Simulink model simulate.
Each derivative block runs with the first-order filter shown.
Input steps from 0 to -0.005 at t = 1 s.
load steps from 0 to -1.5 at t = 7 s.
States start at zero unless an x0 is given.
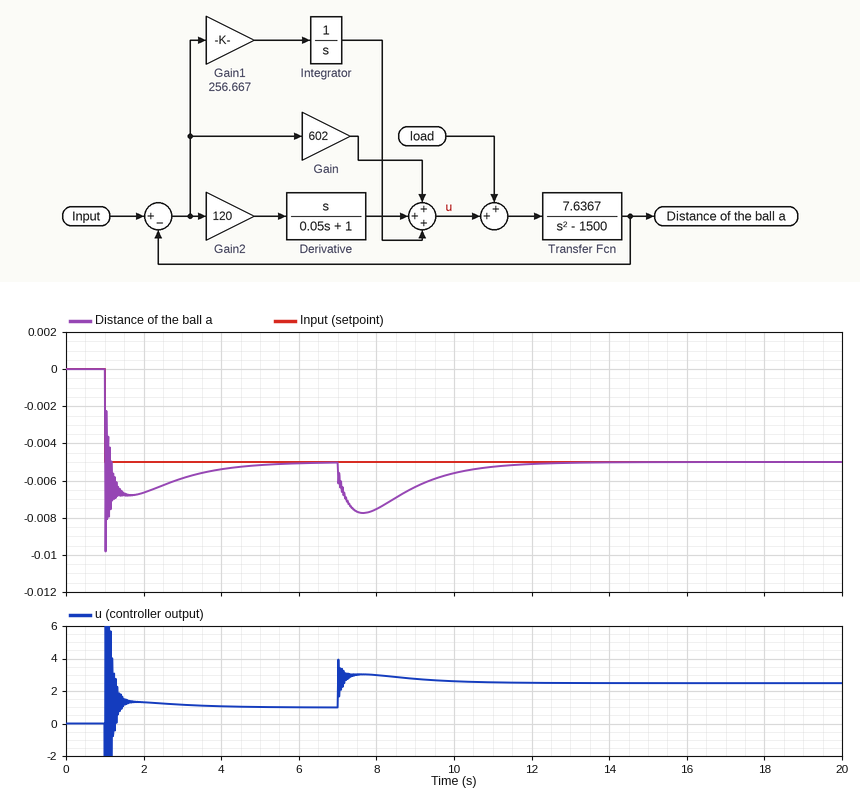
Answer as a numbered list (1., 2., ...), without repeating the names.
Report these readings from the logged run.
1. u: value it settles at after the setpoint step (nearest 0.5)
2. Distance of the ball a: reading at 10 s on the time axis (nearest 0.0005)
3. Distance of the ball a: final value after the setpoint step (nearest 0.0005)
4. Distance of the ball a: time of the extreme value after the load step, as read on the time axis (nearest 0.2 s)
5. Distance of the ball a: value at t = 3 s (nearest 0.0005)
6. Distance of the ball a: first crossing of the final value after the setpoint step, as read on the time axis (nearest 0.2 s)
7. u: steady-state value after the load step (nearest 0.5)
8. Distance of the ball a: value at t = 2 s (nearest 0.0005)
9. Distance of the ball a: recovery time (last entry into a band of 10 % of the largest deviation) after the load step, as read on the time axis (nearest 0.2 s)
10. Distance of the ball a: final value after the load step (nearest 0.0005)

1. 1.0
2. -0.0055
3. -0.0050
4. 7.6 s
5. -0.0060
6. 1.0 s
7. 2.5
8. -0.0065
9. 11.0 s
10. -0.0050
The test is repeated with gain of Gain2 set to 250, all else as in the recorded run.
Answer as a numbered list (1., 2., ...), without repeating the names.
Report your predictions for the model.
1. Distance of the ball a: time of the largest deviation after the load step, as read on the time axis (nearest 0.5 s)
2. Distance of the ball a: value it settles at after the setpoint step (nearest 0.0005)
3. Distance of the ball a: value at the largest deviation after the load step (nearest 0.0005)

1. 8.0 s
2. -0.0050
3. -0.0075
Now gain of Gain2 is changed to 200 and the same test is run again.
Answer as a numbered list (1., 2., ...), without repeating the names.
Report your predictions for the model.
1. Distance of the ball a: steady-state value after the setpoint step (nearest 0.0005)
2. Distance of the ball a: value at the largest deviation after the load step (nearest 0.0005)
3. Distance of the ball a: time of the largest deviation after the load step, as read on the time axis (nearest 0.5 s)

1. -0.0050
2. -0.0075
3. 8.0 s
